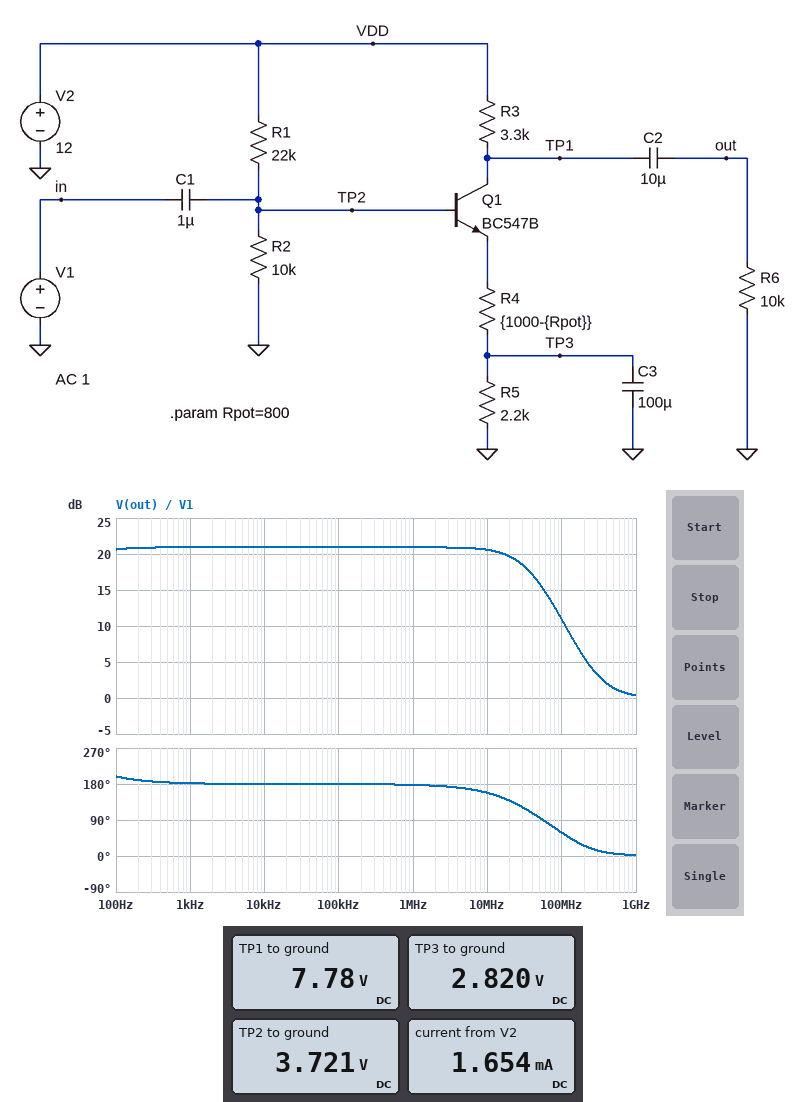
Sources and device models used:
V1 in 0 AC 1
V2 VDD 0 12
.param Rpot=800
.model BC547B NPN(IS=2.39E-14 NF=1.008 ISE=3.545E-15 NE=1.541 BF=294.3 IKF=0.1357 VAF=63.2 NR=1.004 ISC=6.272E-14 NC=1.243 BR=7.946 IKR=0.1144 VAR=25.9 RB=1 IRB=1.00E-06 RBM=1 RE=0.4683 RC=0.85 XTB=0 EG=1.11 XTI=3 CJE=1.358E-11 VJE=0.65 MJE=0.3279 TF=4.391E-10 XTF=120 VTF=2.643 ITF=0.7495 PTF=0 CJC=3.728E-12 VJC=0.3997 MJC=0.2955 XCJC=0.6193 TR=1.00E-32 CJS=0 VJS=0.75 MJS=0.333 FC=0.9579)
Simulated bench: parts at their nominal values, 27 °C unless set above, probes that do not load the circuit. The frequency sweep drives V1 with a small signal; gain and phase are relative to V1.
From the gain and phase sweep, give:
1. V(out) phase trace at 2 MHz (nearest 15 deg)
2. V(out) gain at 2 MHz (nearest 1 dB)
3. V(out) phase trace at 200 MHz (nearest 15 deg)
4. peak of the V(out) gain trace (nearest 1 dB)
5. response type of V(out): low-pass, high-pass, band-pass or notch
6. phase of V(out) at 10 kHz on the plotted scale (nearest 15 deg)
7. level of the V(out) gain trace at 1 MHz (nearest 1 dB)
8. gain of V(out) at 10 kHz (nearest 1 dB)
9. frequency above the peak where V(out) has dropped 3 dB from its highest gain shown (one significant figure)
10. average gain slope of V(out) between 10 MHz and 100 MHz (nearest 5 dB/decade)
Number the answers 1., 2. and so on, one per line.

1. 180 deg
2. 21 dB
3. 30 deg
4. 21 dB
5. low-pass
6. 180 deg
7. 21 dB
8. 21 dB
9. 30 MHz
10. -10 dB/decade
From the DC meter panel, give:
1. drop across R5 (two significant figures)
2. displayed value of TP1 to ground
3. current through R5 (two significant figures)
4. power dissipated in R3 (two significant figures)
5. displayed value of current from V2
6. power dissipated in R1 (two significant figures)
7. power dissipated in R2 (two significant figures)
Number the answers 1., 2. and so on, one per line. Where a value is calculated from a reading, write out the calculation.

1. 2.82 V = 2.8 V
2. 7.78 V
3. (2.82 V) / 2.2 kΩ = 1.3 mA
4. (12 V - 7.78 V)^2 / 3.3 kΩ = 5.4 mW
5. 1.654 mA
6. (12 V - 3.721 V)^2 / 22 kΩ = 3.1 mW
7. (3.721 V)^2 / 10 kΩ = 1.4 mW
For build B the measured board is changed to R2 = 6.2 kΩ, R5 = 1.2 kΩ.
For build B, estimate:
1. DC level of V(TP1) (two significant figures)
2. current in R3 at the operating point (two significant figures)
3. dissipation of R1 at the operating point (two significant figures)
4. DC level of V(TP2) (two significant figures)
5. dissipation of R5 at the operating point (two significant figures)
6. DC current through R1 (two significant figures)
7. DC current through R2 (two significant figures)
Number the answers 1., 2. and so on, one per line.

1. 7.4 V
2. 1.4 mA
3. 4.0 mW
4. 2.6 V
5. 2.4 mW
6. 430 µA
7. 420 µA
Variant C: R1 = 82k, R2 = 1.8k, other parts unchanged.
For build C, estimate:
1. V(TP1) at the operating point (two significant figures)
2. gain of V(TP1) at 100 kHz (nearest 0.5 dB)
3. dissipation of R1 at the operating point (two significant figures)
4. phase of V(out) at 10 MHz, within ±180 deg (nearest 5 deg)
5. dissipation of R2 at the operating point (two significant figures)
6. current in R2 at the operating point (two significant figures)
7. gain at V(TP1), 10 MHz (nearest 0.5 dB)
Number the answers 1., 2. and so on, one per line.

1. 12 V
2. -53.5 dB
3. 1.7 mW
4. 80 deg
5. 37 µW
6. 140 µA
7. -13.5 dB
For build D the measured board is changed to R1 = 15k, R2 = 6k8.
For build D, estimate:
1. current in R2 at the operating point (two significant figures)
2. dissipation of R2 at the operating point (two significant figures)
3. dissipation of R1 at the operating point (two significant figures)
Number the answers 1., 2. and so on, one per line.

1. 550 µA
2. 2.0 mW
3. 4.6 mW
